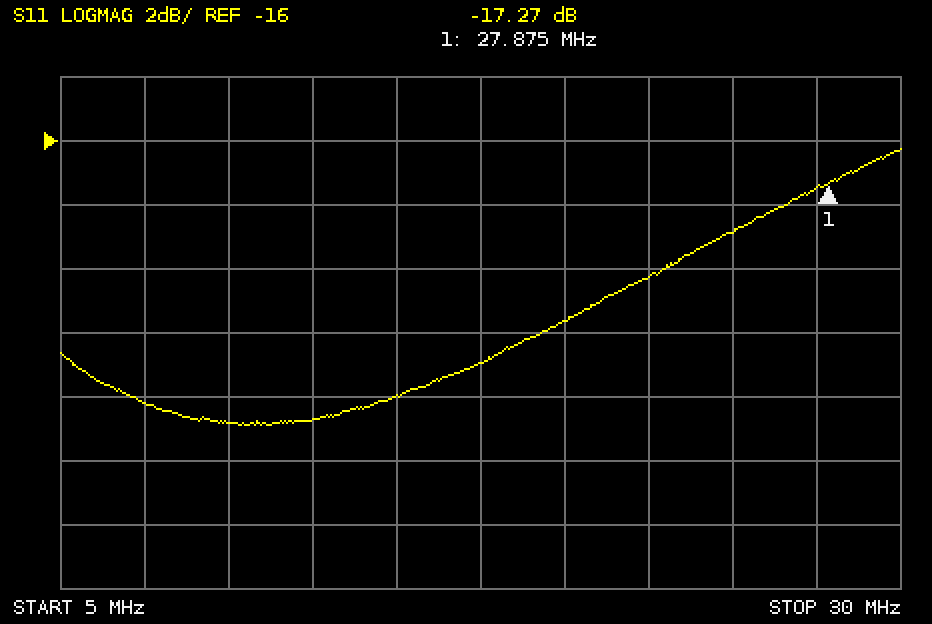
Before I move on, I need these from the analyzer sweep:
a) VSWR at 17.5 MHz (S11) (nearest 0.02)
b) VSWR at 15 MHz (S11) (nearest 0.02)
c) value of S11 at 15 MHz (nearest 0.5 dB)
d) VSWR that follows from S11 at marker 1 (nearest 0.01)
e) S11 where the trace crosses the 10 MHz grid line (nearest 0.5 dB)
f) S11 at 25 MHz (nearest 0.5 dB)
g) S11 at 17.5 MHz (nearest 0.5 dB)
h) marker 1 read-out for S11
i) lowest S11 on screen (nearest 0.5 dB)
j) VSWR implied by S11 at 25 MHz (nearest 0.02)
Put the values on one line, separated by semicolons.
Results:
1.16; 1.14; -24.0 dB; 1.32; -25.0 dB; -19.0 dB; -23.0 dB; -17.27 dB; -25.0 dB; 1.26
